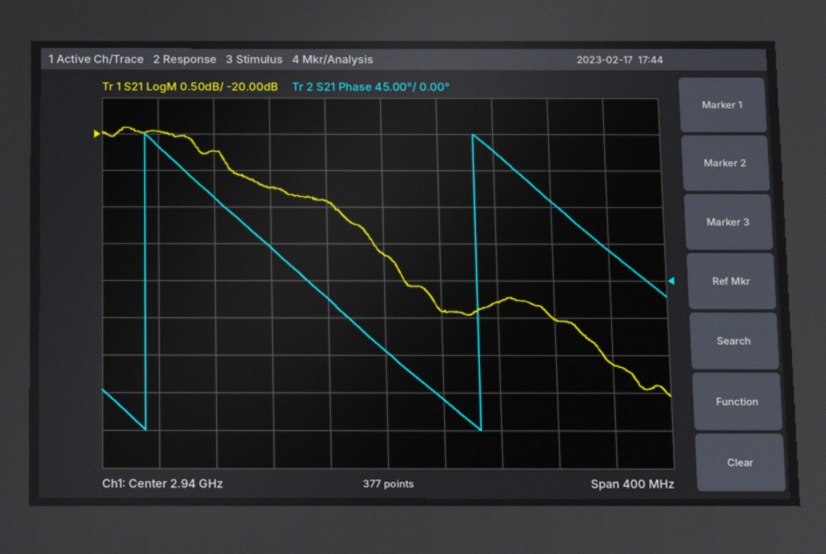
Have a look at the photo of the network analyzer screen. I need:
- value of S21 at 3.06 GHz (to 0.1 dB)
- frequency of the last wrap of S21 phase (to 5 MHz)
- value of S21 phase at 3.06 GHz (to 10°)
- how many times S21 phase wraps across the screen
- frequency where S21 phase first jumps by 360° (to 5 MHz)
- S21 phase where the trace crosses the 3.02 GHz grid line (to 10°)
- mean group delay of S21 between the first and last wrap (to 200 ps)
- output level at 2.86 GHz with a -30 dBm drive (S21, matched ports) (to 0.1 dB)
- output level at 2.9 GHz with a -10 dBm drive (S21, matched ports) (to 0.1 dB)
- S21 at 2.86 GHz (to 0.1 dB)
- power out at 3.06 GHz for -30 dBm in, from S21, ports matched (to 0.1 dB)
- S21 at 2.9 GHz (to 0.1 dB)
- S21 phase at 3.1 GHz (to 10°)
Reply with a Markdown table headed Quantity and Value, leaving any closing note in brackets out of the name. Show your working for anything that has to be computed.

| Quantity | Value |
|---|---|
| value of S21 at 3.06 GHz | -22.5 dB |
| frequency of the last wrap of S21 phase | 3.005 GHz |
| value of S21 phase at 3.06 GHz | 100° |
| how many times S21 phase wraps across the screen | 2 |
| frequency where S21 phase first jumps by 360° | 2.770 GHz |
| S21 phase where the trace crosses the 3.02 GHz grid line | 160° |
| mean group delay of S21 between the first and last wrap | 1 cycle / (3.005 GHz − 2.770 GHz) ≈ 4.26 ns, so 4.2 ns to the nearest 200 ps |
| output level at 2.86 GHz with a -30 dBm drive (S21, matched ports) | -30 dBm + (-20.7 dB) = -50.7 dBm |
| output level at 2.9 GHz with a -10 dBm drive (S21, matched ports) | -10 dBm + (-20.9 dB) = -30.9 dBm |
| S21 at 2.86 GHz | -20.7 dB |
| power out at 3.06 GHz for -30 dBm in, from S21, ports matched | -30 dBm + (-22.5 dB) = -52.5 dBm |
| S21 at 2.9 GHz | -20.9 dB |
| S21 phase at 3.1 GHz | 40° |
